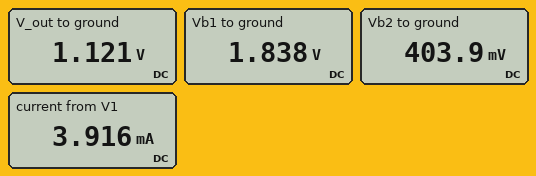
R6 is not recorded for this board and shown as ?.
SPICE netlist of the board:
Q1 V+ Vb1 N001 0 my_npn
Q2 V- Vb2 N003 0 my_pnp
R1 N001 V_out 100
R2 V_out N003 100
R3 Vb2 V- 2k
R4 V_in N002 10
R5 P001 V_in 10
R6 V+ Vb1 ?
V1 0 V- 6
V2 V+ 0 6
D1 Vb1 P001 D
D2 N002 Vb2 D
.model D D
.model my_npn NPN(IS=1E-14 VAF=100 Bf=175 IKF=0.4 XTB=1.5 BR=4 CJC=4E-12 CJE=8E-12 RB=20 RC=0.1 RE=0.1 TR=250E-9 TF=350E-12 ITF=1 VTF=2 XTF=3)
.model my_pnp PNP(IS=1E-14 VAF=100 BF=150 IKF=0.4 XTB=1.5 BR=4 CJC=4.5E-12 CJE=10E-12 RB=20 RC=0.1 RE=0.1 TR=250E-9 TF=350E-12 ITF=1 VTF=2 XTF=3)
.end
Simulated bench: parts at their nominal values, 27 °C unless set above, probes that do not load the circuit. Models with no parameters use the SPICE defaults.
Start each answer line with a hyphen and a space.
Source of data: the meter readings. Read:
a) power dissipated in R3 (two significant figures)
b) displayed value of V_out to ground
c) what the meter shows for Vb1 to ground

- 21 mW
- 1.121 V
- 1.838 V
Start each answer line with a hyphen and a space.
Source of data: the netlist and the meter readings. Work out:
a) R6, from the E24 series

- 1.3 kΩ
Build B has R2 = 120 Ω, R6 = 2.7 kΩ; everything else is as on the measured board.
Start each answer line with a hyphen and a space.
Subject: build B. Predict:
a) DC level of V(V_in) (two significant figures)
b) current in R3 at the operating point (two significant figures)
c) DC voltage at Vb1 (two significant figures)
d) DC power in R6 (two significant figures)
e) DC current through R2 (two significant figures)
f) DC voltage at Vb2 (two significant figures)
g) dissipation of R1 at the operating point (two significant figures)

- -790 mV
- 2.3 mA
- -90 mV
- 14 mW
- 550 µA
- -1.5 V
- 30 µW
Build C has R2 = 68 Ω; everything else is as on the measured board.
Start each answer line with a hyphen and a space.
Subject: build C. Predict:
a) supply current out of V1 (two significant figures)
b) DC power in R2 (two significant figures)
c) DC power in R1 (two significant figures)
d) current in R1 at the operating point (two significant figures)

- 4.0 mA
- 45 µW
- 67 µW
- 820 µA
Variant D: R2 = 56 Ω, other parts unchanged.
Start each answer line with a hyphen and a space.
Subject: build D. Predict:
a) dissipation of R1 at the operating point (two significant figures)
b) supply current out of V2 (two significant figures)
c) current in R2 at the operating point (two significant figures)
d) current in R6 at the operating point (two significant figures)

- 74 µW
- 4.1 mA
- 860 µA
- 3.2 mA
